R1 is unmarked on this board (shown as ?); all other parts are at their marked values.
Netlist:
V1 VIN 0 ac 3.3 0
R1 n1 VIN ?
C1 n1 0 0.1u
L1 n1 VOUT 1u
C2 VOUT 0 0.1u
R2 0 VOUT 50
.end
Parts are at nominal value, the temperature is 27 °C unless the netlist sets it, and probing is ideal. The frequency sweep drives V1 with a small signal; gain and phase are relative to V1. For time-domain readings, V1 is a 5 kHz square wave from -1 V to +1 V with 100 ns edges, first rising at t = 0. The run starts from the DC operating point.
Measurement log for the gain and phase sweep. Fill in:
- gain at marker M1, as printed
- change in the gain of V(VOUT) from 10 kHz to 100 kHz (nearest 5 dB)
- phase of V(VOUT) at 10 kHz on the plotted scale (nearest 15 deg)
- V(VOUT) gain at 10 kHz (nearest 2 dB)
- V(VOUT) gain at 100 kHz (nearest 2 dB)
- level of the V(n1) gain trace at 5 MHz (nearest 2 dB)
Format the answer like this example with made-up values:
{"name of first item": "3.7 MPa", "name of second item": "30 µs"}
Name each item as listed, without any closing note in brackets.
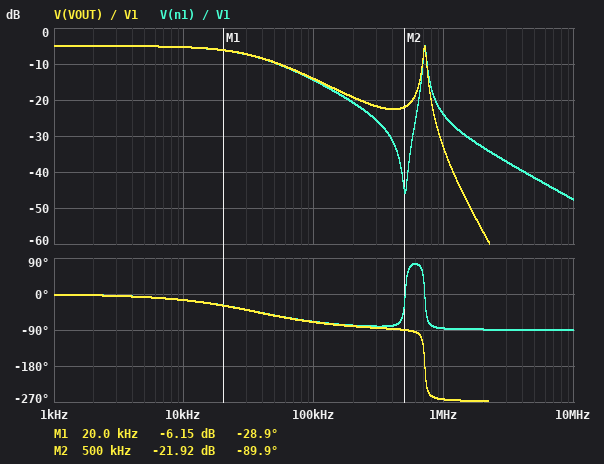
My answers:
{"gain at marker M1, as printed": "-6.15 dB", "change in the gain of V(VOUT) from 10 kHz to 100 kHz": "-10 dB", "phase of V(VOUT) at 10 kHz on the plotted scale": "-15 deg", "V(VOUT) gain at 10 kHz": "-6 dB", "V(VOUT) gain at 100 kHz": "-14 dB", "level of the V(n1) gain trace at 5 MHz": "-42 dB"}
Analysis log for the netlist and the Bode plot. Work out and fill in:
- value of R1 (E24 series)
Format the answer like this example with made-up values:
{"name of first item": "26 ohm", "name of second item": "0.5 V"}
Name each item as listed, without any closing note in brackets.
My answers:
{"value of R1": "39 Ω"}
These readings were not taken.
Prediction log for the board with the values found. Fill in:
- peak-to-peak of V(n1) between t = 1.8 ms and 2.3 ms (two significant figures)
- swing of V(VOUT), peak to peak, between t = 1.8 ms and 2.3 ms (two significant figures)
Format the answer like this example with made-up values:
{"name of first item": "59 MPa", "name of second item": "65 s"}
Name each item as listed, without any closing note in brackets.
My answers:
{"peak-to-peak of V(n1) between t = 1.8 ms and 2.3 ms": "1.1 V", "swing of V(VOUT), peak to peak, between t = 1.8 ms and 2.3 ms": "1.1 V"}
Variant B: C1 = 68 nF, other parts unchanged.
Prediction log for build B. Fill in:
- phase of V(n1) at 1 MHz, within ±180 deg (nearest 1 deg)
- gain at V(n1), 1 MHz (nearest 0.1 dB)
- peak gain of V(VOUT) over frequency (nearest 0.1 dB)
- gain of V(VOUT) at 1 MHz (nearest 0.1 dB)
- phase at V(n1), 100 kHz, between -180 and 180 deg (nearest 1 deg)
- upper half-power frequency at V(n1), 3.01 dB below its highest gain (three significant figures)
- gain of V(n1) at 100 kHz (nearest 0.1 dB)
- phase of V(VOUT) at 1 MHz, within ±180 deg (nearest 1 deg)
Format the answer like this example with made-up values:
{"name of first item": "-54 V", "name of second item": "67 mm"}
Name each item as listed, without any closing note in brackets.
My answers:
{"phase of V(n1) at 1 MHz, within ±180 deg": "-83 deg", "gain at V(n1), 1 MHz": "-18.5 dB", "peak gain of V(VOUT) over frequency": "-5.0 dB", "gain of V(VOUT) at 1 MHz": "-27.9 dB", "phase at V(n1), 100 kHz, between -180 and 180 deg": "-66 deg", "upper half-power frequency at V(n1), 3.01 dB below its highest gain": "818 kHz", "gain of V(n1) at 100 kHz": "-13.2 dB", "phase of V(VOUT) at 1 MHz, within ±180 deg": "100 deg"}
